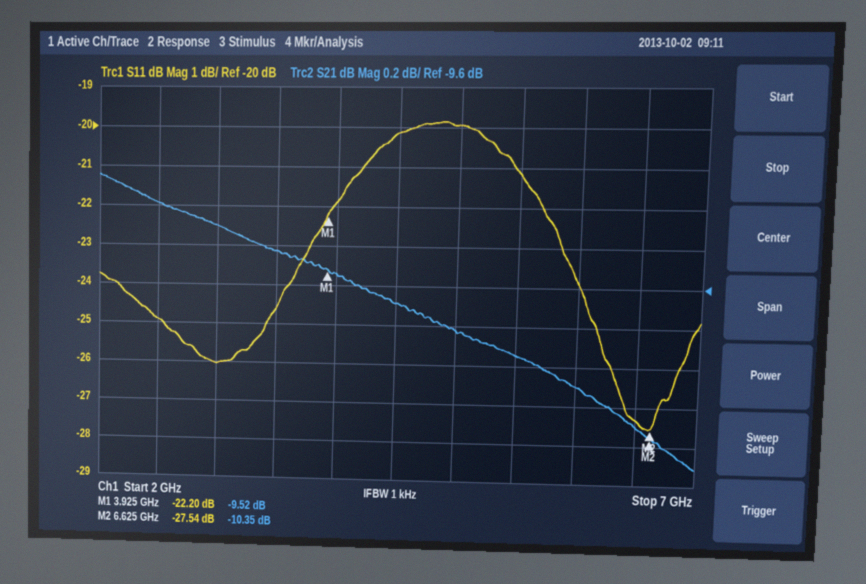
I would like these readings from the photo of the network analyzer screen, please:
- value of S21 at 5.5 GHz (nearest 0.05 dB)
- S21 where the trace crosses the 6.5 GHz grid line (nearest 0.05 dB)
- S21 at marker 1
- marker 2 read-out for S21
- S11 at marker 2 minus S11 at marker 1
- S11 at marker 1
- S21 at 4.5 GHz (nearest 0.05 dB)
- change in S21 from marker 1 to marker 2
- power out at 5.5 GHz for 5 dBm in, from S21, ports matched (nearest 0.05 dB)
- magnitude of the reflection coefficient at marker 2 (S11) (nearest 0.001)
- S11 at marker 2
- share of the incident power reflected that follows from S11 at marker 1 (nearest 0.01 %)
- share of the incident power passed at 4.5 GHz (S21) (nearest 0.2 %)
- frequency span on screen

-9.95 dB
-10.30 dB
-9.52 dB
-10.35 dB
-5.34 dB
-22.20 dB
-9.70 dB
-0.83 dB
-4.95 dBm
0.042
-27.54 dB
0.60 %
10.8 %
5 GHz
